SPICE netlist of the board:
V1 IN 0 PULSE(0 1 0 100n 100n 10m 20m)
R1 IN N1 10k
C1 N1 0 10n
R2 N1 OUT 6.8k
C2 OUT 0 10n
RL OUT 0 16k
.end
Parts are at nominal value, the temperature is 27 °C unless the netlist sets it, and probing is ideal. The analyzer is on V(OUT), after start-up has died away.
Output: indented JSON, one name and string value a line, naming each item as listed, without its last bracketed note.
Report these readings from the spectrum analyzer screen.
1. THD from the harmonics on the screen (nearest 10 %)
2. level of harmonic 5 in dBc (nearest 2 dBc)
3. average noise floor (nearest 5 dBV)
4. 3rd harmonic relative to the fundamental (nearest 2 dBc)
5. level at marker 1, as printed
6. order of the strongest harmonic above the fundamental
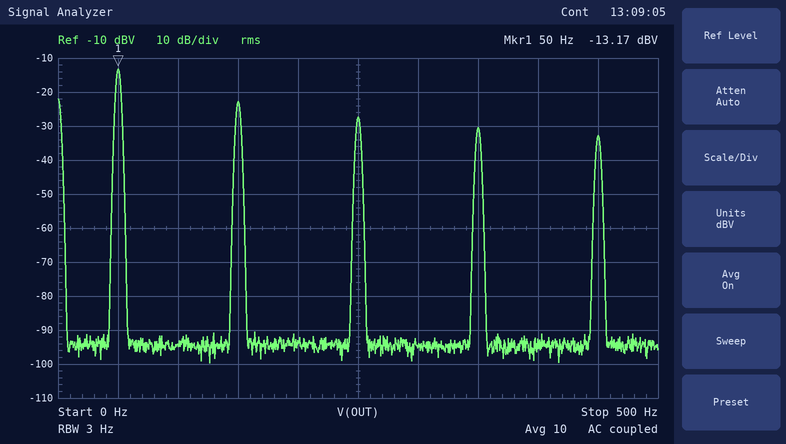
{
  "THD from the harmonics on the screen": "40 %",
  "level of harmonic 5 in dBc": "-14 dBc",
  "average noise floor": "-95 dBV",
  "3rd harmonic relative to the fundamental": "-10 dBc",
  "level at marker 1, as printed": "-13.17 dBV",
  "order of the strongest harmonic above the fundamental": "3"
}
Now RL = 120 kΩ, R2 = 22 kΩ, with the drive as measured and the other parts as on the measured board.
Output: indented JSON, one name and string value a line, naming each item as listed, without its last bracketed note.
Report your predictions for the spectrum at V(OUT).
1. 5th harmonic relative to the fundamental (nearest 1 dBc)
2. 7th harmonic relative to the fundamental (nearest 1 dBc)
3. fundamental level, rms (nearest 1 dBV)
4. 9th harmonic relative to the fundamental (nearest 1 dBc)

{
  "5th harmonic relative to the fundamental": "-15 dBc",
  "7th harmonic relative to the fundamental": "-18 dBc",
  "fundamental level, rms": "-9 dBV",
  "9th harmonic relative to the fundamental": "-21 dBc"
}
